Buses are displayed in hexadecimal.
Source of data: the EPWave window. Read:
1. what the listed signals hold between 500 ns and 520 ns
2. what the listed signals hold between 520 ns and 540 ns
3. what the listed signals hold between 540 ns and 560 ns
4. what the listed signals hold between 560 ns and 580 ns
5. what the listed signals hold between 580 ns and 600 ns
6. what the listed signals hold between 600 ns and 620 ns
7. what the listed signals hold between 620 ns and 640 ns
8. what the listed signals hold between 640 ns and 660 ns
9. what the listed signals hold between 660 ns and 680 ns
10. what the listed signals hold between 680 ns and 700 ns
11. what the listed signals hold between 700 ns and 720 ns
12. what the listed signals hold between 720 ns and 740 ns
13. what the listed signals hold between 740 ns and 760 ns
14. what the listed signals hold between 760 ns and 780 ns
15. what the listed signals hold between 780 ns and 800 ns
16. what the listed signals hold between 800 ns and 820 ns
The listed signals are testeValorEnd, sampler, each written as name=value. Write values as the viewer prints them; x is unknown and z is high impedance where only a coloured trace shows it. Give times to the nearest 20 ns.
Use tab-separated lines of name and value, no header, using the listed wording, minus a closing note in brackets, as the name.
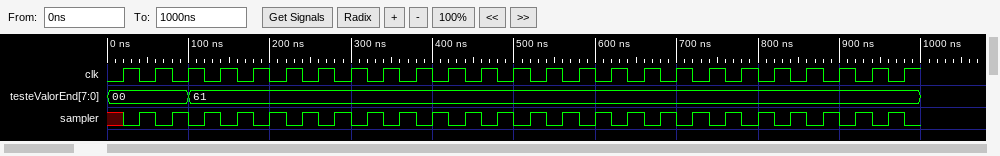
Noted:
what the listed signals hold between 500 ns and 520 ns	testeValorEnd=61, sampler=0
what the listed signals hold between 520 ns and 540 ns	testeValorEnd=61, sampler=1
what the listed signals hold between 540 ns and 560 ns	testeValorEnd=61, sampler=0
what the listed signals hold between 560 ns and 580 ns	testeValorEnd=61, sampler=1
what the listed signals hold between 580 ns and 600 ns	testeValorEnd=61, sampler=0
what the listed signals hold between 600 ns and 620 ns	testeValorEnd=61, sampler=1
what the listed signals hold between 620 ns and 640 ns	testeValorEnd=61, sampler=0
what the listed signals hold between 640 ns and 660 ns	testeValorEnd=61, sampler=1
what the listed signals hold between 660 ns and 680 ns	testeValorEnd=61, sampler=0
what the listed signals hold between 680 ns and 700 ns	testeValorEnd=61, sampler=1
what the listed signals hold between 700 ns and 720 ns	testeValorEnd=61, sampler=0
what the listed signals hold between 720 ns and 740 ns	testeValorEnd=61, sampler=1
what the listed signals hold between 740 ns and 760 ns	testeValorEnd=61, sampler=0
what the listed signals hold between 760 ns and 780 ns	testeValorEnd=61, sampler=1
what the listed signals hold between 780 ns and 800 ns	testeValorEnd=61, sampler=0
what the listed signals hold between 800 ns and 820 ns	testeValorEnd=61, sampler=1
